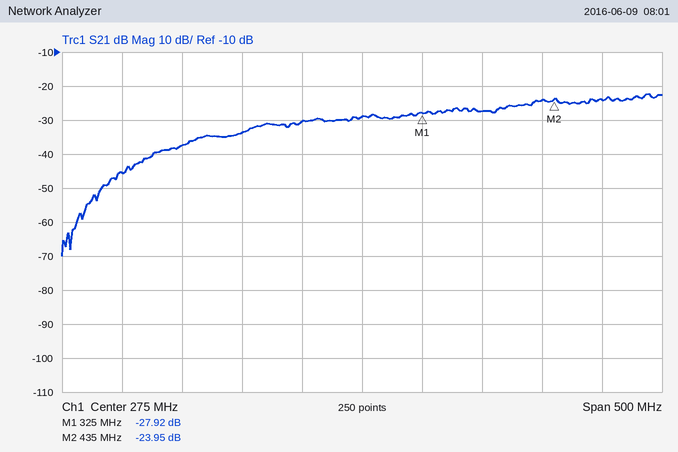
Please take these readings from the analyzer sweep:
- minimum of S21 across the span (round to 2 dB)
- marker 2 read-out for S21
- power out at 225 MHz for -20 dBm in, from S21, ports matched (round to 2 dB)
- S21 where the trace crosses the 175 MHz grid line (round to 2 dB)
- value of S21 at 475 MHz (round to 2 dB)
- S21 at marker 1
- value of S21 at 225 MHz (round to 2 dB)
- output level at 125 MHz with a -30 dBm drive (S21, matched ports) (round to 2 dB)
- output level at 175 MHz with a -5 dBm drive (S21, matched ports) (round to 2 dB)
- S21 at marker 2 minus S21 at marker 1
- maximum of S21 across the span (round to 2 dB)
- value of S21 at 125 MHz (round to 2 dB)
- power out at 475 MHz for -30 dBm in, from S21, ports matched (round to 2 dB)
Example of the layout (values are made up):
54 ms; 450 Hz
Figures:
-70 dB; -23.95 dB; -50 dBm; -34 dB; -24 dB; -27.92 dB; -30 dB; -68 dBm; -38 dBm; 3.97 dB; -22 dB; -38 dB; -54 dBm
